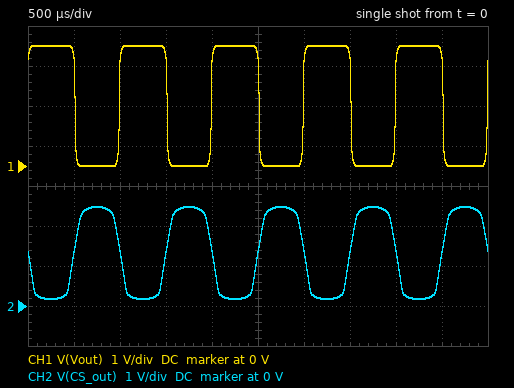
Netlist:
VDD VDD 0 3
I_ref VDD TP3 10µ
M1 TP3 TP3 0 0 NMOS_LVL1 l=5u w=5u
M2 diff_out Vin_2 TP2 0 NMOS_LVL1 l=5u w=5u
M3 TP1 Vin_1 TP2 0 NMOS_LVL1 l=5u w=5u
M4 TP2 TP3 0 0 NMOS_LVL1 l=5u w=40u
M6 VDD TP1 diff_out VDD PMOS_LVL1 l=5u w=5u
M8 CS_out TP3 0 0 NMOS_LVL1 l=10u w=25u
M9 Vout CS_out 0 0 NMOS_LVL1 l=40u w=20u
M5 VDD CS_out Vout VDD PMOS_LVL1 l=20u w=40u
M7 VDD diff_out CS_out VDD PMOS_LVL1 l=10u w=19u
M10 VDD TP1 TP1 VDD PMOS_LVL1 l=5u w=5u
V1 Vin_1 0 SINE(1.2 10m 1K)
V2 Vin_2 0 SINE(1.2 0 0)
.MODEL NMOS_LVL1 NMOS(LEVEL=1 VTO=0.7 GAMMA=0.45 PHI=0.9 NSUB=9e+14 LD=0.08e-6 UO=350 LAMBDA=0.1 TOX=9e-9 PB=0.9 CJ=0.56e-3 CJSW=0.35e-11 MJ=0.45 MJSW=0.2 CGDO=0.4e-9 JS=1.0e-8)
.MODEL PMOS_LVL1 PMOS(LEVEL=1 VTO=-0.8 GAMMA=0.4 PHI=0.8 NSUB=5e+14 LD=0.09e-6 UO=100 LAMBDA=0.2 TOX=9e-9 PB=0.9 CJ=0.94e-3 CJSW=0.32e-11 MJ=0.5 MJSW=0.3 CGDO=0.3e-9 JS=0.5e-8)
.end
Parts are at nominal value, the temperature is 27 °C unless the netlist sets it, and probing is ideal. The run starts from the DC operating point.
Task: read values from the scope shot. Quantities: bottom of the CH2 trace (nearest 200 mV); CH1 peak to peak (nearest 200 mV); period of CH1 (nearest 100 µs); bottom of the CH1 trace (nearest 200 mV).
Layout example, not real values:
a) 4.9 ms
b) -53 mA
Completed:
a) 200 mV
b) 3.0 V
c) 1.0 ms
d) 0 V
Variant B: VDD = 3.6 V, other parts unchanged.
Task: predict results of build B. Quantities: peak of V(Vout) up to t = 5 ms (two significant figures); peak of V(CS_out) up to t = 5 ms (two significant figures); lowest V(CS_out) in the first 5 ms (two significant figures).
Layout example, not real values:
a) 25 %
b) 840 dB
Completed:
a) 3.6 V
b) 3.1 V
c) 190 mV
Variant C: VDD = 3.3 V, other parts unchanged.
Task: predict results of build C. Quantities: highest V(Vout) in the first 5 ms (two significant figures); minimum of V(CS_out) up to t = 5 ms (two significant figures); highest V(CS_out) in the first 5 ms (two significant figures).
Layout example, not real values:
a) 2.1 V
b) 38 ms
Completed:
a) 3.3 V
b) 180 mV
c) 2.8 V
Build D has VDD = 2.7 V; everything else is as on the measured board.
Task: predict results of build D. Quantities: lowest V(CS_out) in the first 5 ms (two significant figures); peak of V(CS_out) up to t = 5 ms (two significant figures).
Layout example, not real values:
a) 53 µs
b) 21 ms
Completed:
a) 160 mV
b) 2.2 V
